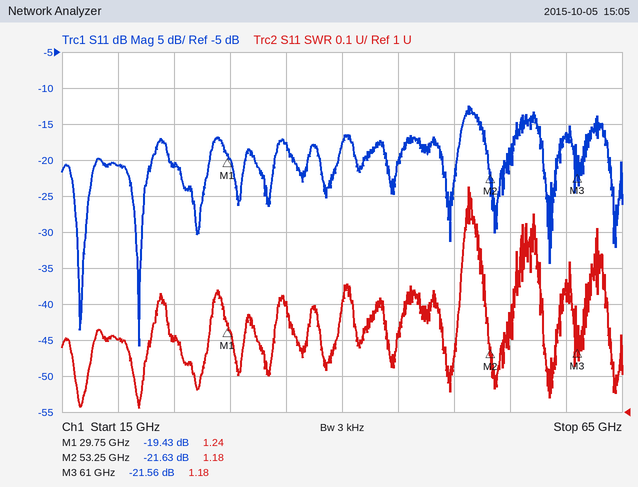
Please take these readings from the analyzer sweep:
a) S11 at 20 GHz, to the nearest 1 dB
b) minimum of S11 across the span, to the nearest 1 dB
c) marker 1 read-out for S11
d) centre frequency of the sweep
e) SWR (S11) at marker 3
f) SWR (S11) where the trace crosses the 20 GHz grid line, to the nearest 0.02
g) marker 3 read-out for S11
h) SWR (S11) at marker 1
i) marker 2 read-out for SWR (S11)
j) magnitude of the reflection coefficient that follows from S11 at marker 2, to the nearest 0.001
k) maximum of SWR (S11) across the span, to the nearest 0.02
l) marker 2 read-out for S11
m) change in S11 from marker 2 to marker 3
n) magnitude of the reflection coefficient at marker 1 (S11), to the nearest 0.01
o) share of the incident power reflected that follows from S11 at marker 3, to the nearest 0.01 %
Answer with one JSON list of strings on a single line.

["-21 dB", "-46 dB", "-19.43 dB", "40 GHz", "1.18", "1.20", "-21.56 dB", "1.24", "1.18", "0.083", "1.62", "-21.63 dB", "0.07 dB", "0.11", "0.70 %"]
